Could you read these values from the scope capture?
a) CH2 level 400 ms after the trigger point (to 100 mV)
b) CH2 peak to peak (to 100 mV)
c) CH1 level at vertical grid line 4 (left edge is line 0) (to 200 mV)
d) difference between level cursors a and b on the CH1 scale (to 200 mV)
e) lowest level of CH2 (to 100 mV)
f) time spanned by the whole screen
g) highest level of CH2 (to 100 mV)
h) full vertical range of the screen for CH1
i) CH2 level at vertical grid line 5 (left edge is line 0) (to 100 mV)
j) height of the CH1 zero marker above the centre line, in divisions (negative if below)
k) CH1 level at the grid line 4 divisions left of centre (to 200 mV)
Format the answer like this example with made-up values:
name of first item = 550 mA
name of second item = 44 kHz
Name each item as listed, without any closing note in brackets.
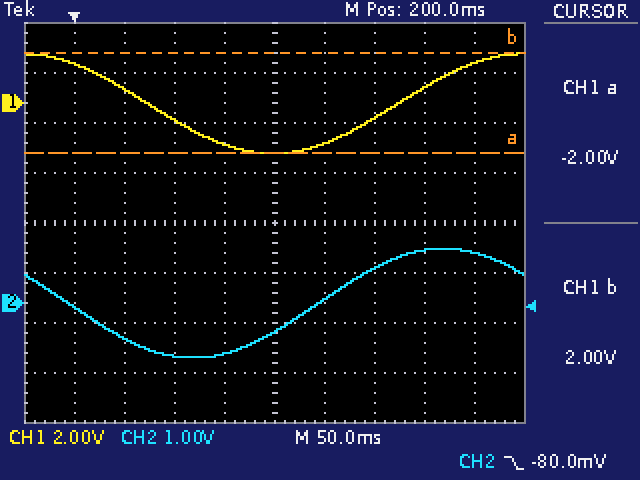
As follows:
CH2 level 400 ms after the trigger point = 1.0 V
CH2 peak to peak = 2.2 V
CH1 level at vertical grid line 4 (left edge is line 0) = -1.6 V
difference between level cursors a and b on the CH1 scale = 4.0 V
lowest level of CH2 = -1.1 V
time spanned by the whole screen = 500 ms
highest level of CH2 = 1.1 V
full vertical range of the screen for CH1 = 16 V
CH2 level at vertical grid line 5 (left edge is line 0) = -600 mV
height of the CH1 zero marker above the centre line, in divisions = +2.4 div
CH1 level at the grid line 4 divisions left of centre = 1.6 V
